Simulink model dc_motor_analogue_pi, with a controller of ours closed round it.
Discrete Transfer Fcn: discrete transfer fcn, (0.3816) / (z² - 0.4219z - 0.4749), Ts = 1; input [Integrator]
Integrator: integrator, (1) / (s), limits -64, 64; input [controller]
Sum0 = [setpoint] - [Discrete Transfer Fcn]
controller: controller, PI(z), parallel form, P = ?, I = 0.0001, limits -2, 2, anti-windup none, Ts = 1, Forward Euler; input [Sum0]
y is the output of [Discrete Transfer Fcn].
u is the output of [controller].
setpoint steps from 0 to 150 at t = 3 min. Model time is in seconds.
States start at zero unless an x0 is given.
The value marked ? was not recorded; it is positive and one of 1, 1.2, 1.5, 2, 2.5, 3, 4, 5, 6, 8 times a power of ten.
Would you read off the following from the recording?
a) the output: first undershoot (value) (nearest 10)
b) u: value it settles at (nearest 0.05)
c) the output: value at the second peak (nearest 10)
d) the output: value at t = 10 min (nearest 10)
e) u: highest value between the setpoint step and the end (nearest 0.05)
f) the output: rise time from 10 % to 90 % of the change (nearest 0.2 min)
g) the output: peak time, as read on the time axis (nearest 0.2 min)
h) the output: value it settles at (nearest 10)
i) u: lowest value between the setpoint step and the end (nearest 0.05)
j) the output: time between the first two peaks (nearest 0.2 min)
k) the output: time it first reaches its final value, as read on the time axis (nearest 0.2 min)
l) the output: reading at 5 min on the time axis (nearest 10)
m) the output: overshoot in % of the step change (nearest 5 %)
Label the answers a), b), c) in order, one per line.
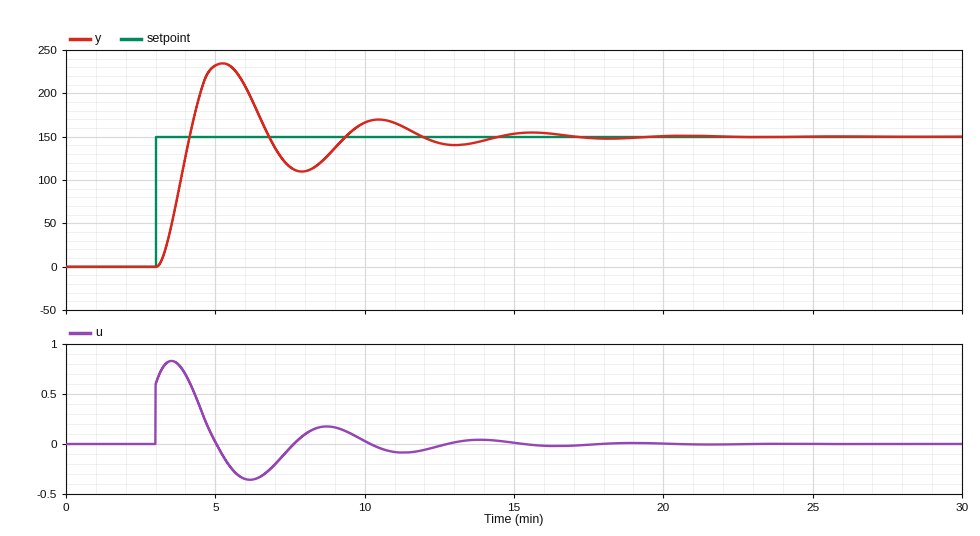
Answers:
a) 110
b) 0.00
c) 170
d) 170
e) 0.85
f) 0.8 min
g) 5.2 min
h) 150
i) -0.35
j) 5.2 min
k) 4.2 min
l) 230
m) 55 %
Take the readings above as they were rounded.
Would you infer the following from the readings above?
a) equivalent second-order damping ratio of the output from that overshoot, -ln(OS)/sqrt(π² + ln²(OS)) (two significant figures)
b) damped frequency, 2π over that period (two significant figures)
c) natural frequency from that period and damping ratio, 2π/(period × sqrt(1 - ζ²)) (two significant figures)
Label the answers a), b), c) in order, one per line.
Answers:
a) 0.19
b) 1.2 rad/min
c) 1.2 rad/min
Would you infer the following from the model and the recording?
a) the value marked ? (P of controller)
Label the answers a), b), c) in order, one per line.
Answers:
a) 0.004
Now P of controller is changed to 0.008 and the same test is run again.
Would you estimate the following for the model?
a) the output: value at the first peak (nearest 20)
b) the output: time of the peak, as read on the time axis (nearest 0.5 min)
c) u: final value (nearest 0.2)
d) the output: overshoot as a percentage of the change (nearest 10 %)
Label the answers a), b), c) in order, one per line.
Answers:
a) 200
b) 4.5 min
c) 0.0
d) 40 %
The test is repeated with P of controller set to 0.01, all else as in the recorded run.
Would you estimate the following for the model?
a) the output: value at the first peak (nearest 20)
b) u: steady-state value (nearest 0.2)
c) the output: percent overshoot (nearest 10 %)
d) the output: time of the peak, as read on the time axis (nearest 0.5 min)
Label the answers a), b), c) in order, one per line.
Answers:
a) 200
b) 0.0
c) 30 %
d) 4.5 min
